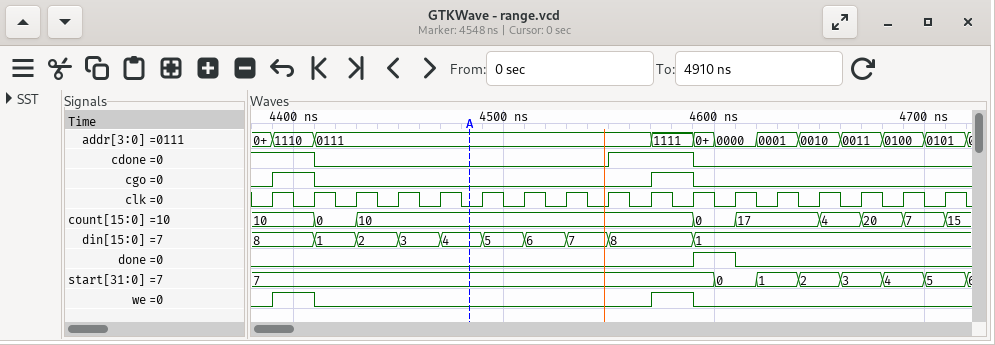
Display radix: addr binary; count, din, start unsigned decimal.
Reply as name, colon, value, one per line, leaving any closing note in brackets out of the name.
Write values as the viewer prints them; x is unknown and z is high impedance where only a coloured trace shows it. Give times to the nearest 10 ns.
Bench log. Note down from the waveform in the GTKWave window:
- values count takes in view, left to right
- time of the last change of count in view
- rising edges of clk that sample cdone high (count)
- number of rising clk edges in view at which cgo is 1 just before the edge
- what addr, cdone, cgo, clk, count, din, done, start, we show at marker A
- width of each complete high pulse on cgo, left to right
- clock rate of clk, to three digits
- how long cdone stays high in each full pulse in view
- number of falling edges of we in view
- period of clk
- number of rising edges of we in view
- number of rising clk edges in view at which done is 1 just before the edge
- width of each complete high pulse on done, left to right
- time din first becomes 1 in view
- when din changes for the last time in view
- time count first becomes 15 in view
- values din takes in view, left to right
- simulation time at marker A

values count takes in view, left to right: 10, 0, 10, 0, 17, 4, 20, 7, 15
time of the last change of count in view: 4710 ns
rising edges of clk that sample cdone high: 4
number of rising clk edges in view at which cgo is 1 just before the edge: 2
what addr, cdone, cgo, clk, count, din, done, start, we show at marker A: addr=0111, cdone=0, cgo=0, clk=0, count=10, din=4, done=0, start=7, we=0
width of each complete high pulse on cgo, left to right: 20 ns, 20 ns
clock rate of clk, to three digits: 50.0 MHz
how long cdone stays high in each full pulse in view: 40 ns
number of falling edges of we in view: 2
period of clk: 20 ns
number of rising edges of we in view: 2
number of rising clk edges in view at which done is 1 just before the edge: 1
width of each complete high pulse on done, left to right: 20 ns
time din first becomes 1 in view: 4410 ns
when din changes for the last time in view: 4590 ns
time count first becomes 15 in view: 4710 ns
values din takes in view, left to right: 8, 1, 2, 3, 4, 5, 6, 7, 8, 1
simulation time at marker A: 4480 ns
